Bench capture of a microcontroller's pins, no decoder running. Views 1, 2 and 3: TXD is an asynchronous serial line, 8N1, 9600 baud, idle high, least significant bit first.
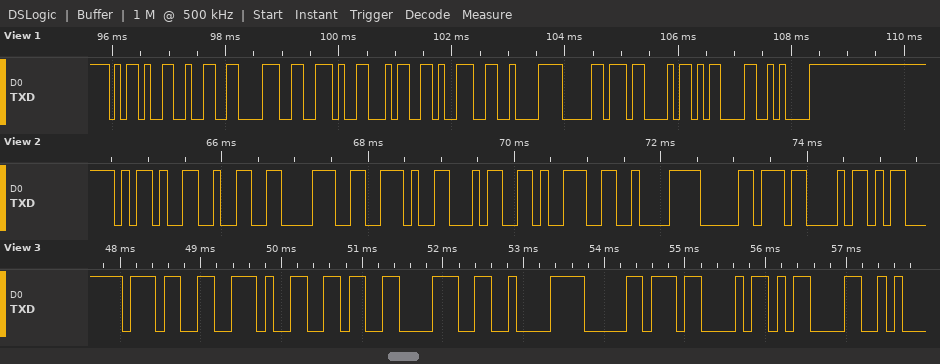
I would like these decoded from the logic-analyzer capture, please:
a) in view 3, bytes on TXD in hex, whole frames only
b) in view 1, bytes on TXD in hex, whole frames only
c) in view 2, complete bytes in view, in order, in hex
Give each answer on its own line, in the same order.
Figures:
37 2E 36 38 C2 B0 43 0D
2D 32 38 2E 34 39 C2 B0 43 0D 0A
2D 32 38 2E 34 39 C2 B0 43
